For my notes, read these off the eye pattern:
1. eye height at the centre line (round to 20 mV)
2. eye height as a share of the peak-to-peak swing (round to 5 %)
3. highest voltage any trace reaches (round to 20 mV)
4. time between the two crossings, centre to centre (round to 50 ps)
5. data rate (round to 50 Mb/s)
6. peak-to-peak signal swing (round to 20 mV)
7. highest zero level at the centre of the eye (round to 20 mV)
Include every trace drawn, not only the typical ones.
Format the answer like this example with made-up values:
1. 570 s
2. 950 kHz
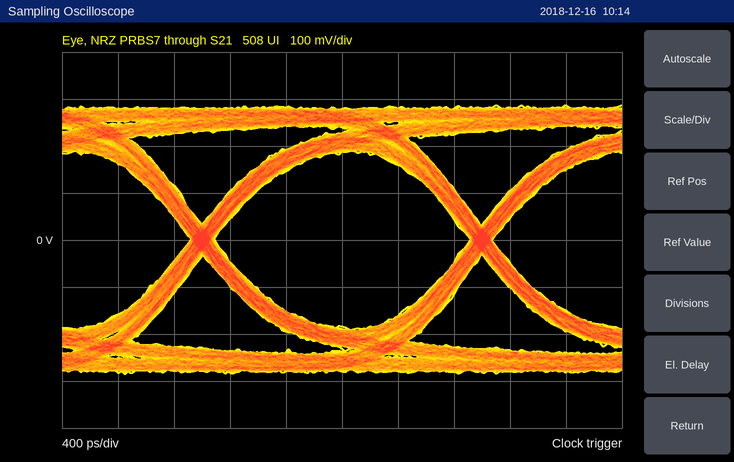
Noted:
1. 380 mV
2. 65 %
3. 280 mV
4. 2.00 ns
5. 500 Mb/s
6. 580 mV
7. -180 mV
